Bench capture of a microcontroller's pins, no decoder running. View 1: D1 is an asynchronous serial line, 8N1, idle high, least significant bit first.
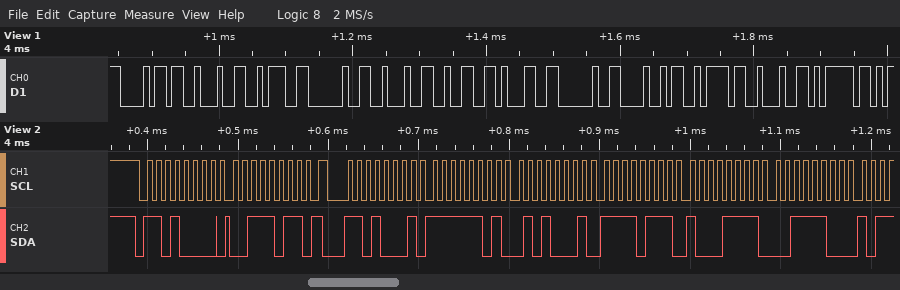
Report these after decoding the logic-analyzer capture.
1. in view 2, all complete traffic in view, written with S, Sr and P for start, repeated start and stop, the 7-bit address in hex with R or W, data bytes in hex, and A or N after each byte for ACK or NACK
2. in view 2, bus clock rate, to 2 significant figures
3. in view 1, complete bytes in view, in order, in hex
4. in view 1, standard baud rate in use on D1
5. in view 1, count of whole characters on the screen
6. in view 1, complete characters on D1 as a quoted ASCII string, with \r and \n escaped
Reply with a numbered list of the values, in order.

1. S 68W A 3B A Sr 68R A FD A 51 A F7 A 8F A 3C A
2. 100 kHz
3. 68 22 3A 20 22 32 31 20 48 7A 22 7D
4. 115200 baud
5. 12
6. "h\": \"21 Hz\"}"
